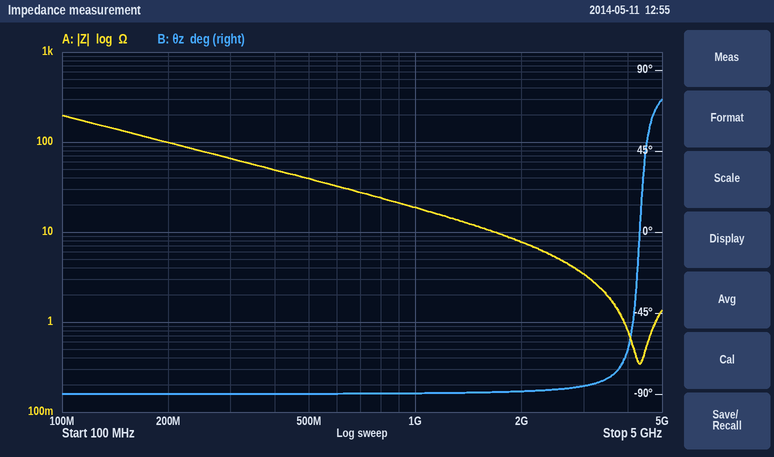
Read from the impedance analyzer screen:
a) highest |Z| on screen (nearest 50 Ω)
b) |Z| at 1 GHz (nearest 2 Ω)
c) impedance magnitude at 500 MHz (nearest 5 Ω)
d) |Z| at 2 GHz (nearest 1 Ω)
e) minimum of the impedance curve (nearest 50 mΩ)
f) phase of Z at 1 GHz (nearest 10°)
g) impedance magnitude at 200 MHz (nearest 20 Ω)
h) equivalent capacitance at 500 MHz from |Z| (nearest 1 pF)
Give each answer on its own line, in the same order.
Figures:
200 Ω
18 Ω
40 Ω
8 Ω
350 mΩ
-90°
100 Ω
8 pF
